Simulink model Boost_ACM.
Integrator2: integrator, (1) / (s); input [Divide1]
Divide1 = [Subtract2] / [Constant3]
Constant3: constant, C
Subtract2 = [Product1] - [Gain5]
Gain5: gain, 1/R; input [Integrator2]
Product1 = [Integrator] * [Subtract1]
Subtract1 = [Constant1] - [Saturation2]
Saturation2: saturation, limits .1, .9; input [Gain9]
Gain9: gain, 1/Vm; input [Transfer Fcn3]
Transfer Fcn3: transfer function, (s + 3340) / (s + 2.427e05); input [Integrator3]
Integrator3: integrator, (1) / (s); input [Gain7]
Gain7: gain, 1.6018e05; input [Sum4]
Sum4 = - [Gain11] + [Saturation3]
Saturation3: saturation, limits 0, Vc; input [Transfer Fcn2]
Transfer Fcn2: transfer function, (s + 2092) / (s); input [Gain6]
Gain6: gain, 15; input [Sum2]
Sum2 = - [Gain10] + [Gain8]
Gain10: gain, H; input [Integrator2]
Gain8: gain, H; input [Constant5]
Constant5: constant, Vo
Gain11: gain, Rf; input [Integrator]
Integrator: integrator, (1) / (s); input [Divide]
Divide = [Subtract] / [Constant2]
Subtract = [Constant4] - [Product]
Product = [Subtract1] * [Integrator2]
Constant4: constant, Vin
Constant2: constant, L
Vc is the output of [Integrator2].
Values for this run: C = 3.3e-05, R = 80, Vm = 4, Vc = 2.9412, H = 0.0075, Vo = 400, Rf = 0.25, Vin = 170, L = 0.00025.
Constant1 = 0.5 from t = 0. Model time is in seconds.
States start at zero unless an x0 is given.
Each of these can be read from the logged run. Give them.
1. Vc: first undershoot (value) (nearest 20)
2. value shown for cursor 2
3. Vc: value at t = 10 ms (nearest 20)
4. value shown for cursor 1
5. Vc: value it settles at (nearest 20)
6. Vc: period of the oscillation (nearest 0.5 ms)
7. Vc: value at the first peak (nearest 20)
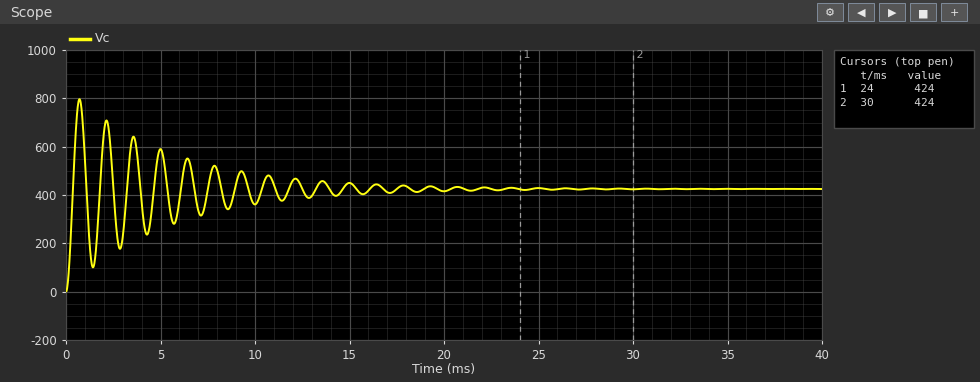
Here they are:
100
424
360
424
420
1.5 ms
800
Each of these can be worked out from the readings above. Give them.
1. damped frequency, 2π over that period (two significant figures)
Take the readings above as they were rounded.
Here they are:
4.2 rad/ms
